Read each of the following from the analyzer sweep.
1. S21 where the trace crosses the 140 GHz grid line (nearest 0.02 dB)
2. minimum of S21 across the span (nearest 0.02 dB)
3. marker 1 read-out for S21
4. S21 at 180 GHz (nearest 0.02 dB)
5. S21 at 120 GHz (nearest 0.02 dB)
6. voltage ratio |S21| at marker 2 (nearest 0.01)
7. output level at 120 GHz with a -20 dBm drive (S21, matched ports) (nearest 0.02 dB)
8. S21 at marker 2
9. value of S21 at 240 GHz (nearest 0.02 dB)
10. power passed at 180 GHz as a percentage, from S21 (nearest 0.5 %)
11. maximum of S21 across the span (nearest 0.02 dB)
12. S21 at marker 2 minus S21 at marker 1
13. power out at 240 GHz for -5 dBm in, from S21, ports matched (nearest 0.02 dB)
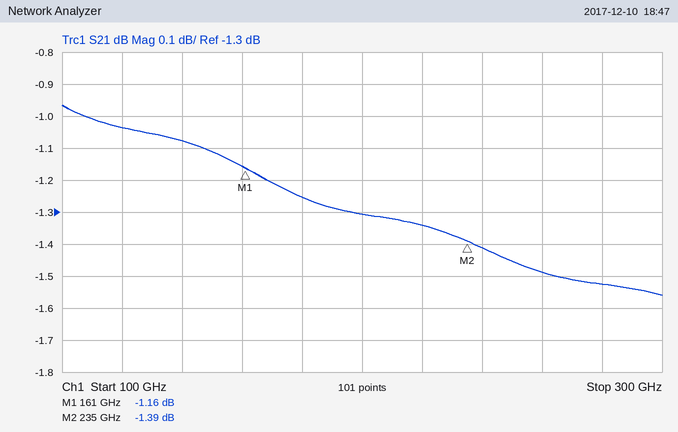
-1.08 dB
-1.56 dB
-1.16 dB
-1.26 dB
-1.04 dB
0.85
-21.04 dBm
-1.39 dB
-1.42 dB
75.0 %
-0.96 dB
-0.23 dB
-6.42 dBm
